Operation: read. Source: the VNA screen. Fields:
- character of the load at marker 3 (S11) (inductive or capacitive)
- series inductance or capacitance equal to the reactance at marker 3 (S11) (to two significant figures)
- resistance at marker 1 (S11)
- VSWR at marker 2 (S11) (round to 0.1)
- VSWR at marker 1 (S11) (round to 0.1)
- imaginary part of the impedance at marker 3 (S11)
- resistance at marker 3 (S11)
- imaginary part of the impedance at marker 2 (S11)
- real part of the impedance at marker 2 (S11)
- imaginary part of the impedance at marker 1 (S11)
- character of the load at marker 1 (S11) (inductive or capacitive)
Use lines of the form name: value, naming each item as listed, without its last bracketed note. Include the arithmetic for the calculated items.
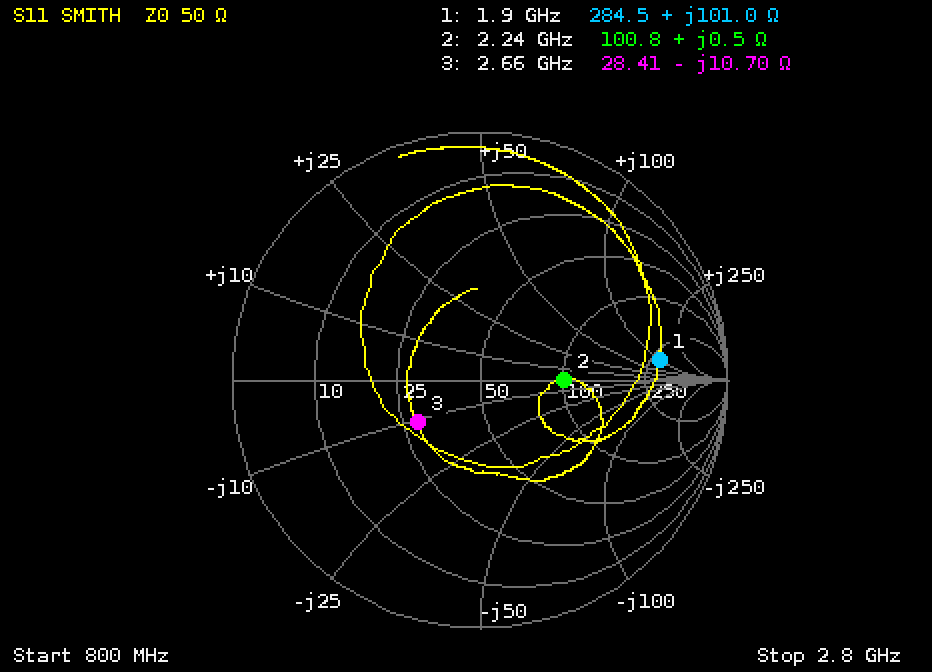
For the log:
character of the load at marker 3 (S11): capacitive
series inductance or capacitance equal to the reactance at marker 3 (S11): C = 1/(2π × 2.66 GHz × 10.7 Ω) ≈ 5.6 pF
resistance at marker 1: 284.5 Ω
VSWR at marker 2 (S11): 2.0
VSWR at marker 1 (S11): 6.4
imaginary part of the impedance at marker 3: -10.70 Ω
resistance at marker 3: 28.41 Ω
imaginary part of the impedance at marker 2: +0.5 Ω
real part of the impedance at marker 2: 100.8 Ω
imaginary part of the impedance at marker 1: +101.0 Ω
character of the load at marker 1 (S11): inductive
